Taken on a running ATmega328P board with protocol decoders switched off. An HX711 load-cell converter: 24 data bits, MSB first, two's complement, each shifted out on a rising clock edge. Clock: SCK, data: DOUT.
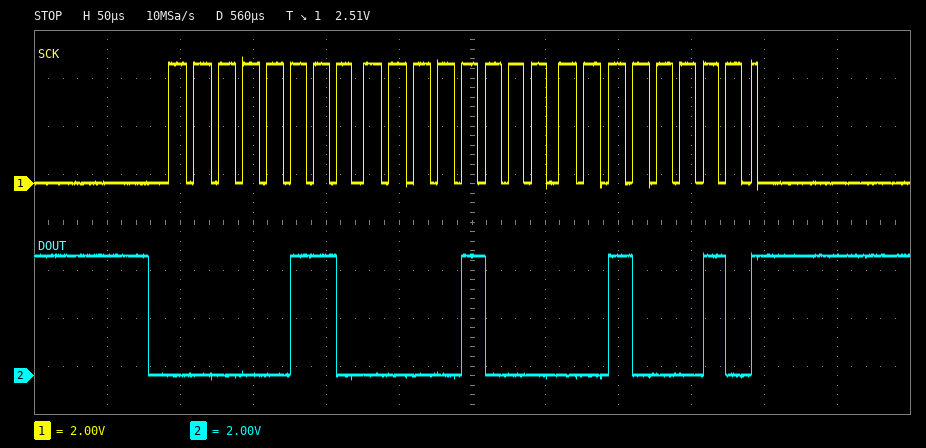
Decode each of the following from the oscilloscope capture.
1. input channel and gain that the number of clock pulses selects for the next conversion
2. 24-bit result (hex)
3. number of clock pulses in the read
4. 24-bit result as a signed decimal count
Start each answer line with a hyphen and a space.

- channel A, gain 128
- 0x060822
- 25
- 395298
